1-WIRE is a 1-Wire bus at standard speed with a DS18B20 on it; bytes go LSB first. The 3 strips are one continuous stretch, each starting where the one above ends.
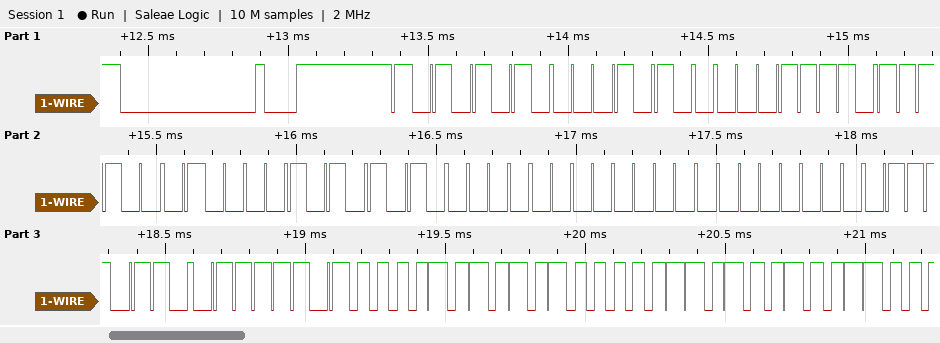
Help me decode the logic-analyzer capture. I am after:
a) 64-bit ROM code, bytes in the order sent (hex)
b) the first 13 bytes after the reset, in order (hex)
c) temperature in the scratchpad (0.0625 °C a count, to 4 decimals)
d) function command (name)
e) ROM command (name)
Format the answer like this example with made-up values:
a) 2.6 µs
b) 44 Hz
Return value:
a) 28 78 8F 50 05 00 00 6E
b) 55 28 78 8F 50 05 00 00 6E BE 50 05 4B
c) 85.0000 °C
d) Read Scratchpad
e) Match ROM
